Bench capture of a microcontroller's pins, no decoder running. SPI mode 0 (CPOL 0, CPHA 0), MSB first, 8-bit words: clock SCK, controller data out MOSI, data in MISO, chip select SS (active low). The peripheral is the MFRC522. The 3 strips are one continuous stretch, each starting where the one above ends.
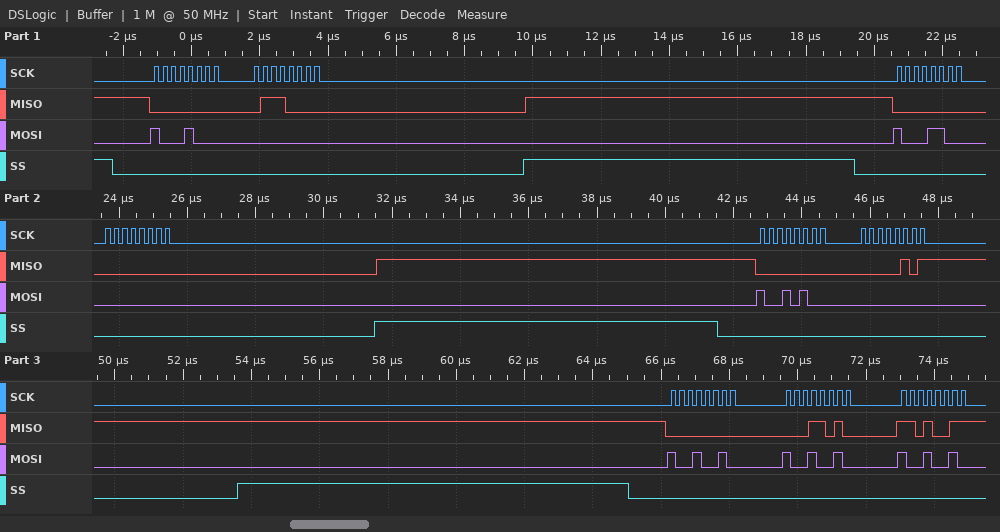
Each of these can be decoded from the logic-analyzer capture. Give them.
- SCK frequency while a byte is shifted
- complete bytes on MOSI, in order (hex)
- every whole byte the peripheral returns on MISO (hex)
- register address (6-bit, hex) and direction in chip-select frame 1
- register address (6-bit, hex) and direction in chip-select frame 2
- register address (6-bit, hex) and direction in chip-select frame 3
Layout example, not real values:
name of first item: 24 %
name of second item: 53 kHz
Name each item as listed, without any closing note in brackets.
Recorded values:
SCK frequency while a byte is shifted: 4 MHz
complete bytes on MOSI, in order: 88 00 8C 00 94 00 92 92 92
every whole byte the peripheral returns on MISO: 00 70 00 00 00 05 00 1A D3
register address (6-bit, hex) and direction in chip-select frame 1: 0x04 read
register address (6-bit, hex) and direction in chip-select frame 2: 0x06 read
register address (6-bit, hex) and direction in chip-select frame 3: 0x0A read
